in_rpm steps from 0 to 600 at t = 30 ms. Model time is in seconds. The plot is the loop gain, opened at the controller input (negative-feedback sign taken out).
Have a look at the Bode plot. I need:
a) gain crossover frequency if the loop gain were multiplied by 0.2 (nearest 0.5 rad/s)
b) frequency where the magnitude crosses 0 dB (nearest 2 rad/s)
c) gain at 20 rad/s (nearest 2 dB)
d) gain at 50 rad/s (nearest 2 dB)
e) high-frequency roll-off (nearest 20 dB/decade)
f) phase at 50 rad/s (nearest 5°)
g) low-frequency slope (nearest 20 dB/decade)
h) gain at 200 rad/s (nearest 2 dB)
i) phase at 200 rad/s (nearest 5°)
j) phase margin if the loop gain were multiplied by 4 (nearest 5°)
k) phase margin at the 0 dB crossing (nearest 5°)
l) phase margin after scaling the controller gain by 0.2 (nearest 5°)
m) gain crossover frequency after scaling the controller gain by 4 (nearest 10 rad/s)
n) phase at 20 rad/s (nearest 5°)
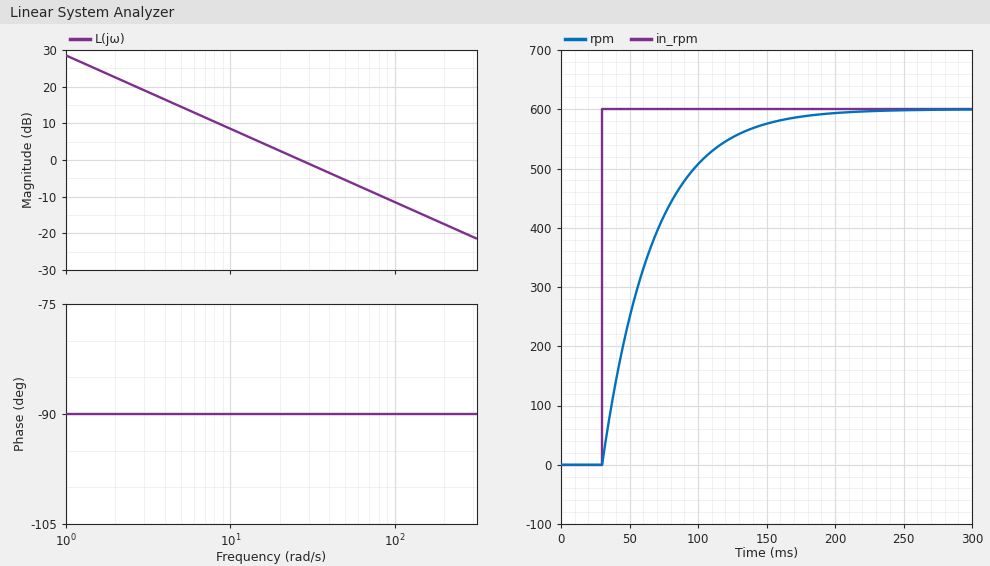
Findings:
5.5 rad/s
26 rad/s
2 dB
-6 dB
-20 dB/decade
-90°
-20 dB/decade
-18 dB
-90°
90°
90°
90°
110 rad/s
-90°
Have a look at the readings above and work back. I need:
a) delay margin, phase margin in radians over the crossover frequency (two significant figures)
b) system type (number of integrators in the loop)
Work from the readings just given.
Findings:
0.060 s
1
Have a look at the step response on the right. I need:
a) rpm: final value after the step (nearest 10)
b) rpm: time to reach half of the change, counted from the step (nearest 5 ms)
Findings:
600
25 ms
